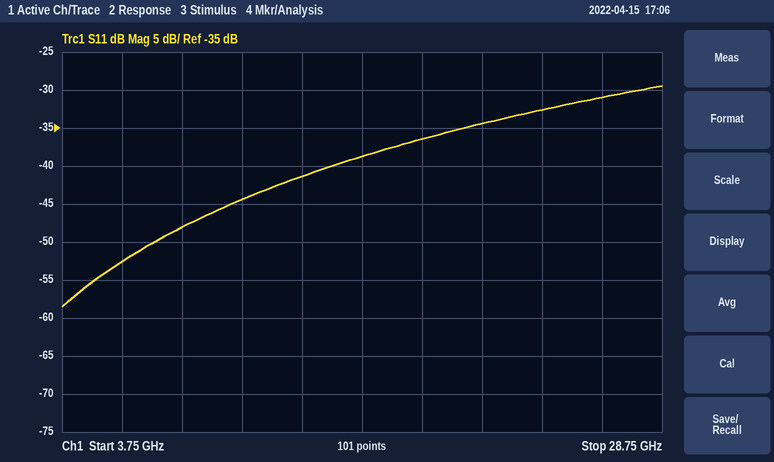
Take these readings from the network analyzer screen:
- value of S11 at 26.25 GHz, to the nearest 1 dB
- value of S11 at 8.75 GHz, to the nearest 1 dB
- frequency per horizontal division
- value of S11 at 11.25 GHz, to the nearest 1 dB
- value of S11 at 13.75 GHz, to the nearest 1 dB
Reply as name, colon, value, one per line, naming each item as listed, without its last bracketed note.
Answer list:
value of S11 at 26.25 GHz, to the nearest 1 dB: -31 dB
value of S11 at 8.75 GHz, to the nearest 1 dB: -48 dB
frequency per horizontal division: 2.5 GHz
value of S11 at 11.25 GHz, to the nearest 1 dB: -44 dB
value of S11 at 13.75 GHz, to the nearest 1 dB: -41 dB
